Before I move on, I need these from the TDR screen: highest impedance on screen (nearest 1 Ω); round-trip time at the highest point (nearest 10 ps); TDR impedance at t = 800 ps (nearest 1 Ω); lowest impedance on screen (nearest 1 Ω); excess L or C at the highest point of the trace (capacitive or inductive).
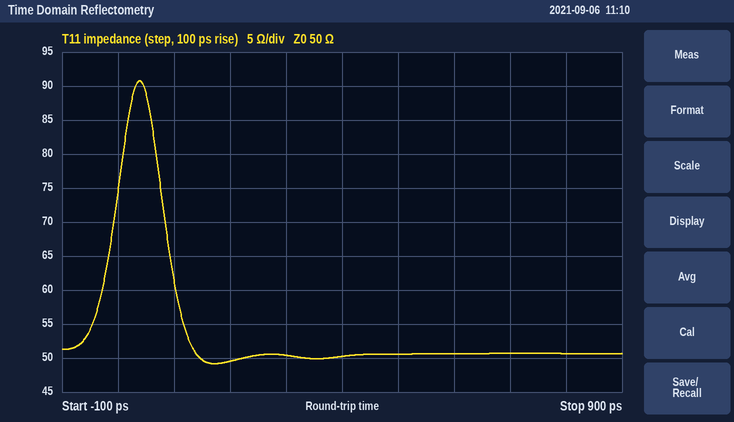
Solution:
91 Ω
40 ps
51 Ω
49 Ω
inductive
